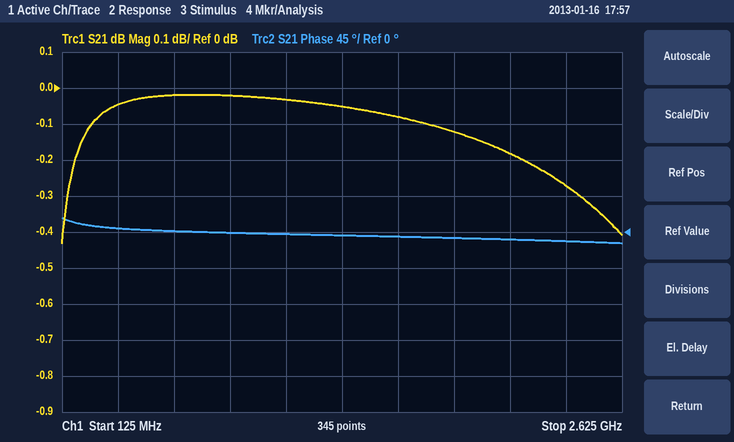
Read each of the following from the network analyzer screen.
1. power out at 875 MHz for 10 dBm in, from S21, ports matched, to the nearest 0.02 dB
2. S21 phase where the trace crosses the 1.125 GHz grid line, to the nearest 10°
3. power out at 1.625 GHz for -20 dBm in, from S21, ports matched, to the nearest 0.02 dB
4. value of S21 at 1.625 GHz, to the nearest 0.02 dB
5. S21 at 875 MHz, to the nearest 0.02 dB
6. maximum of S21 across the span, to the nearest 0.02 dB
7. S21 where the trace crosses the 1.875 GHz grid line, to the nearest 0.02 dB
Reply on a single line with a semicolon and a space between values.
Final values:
9.98 dBm; 0°; -20.08 dBm; -0.08 dB; -0.02 dB; -0.02 dB; -0.12 dB
